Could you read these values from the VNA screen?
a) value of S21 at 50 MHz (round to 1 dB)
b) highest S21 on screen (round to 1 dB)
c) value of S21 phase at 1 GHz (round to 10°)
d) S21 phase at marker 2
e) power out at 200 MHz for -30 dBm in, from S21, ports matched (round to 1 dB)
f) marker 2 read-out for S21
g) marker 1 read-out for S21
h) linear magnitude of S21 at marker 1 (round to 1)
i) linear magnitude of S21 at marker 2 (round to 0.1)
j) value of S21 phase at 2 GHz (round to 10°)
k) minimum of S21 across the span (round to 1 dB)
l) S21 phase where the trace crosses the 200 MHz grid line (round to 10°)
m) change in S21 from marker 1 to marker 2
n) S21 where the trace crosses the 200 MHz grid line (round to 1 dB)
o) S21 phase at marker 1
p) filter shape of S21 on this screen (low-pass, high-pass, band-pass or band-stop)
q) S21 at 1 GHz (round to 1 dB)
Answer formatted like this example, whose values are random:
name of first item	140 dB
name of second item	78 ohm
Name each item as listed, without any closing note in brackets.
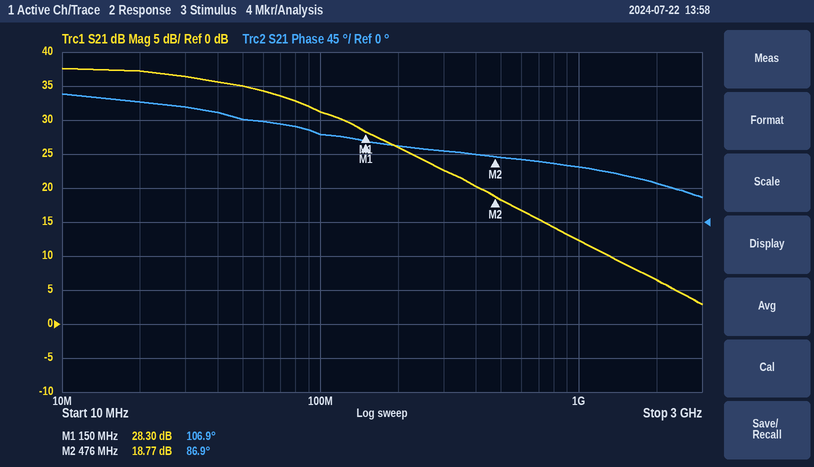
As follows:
value of S21 at 50 MHz	35 dB
highest S21 on screen	38 dB
value of S21 phase at 1 GHz	70°
S21 phase at marker 2	86.9°
power out at 200 MHz for -30 dBm in, from S21, ports matched	-4 dBm
marker 2 read-out for S21	18.77 dB
marker 1 read-out for S21	28.30 dB
linear magnitude of S21 at marker 1	26
linear magnitude of S21 at marker 2	8.7
value of S21 phase at 2 GHz	50°
minimum of S21 across the span	3 dB
S21 phase where the trace crosses the 200 MHz grid line	100°
change in S21 from marker 1 to marker 2	-9.53 dB
S21 where the trace crosses the 200 MHz grid line	26 dB
S21 phase at marker 1	106.9°
filter shape of S21 on this screen	low-pass
S21 at 1 GHz	12 dB
